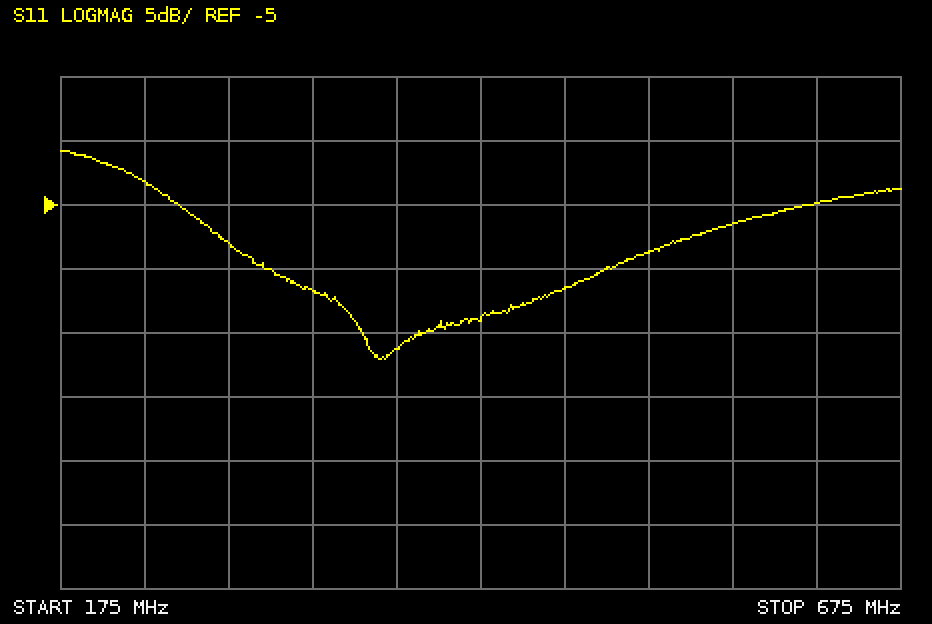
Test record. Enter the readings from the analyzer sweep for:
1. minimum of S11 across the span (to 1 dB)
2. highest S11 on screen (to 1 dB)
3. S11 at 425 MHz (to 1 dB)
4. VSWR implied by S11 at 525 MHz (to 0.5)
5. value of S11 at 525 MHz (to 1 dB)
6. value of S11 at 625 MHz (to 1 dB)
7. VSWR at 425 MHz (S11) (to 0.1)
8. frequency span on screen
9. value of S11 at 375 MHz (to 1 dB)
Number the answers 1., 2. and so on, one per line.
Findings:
1. -17 dB
2. -1 dB
3. -14 dB
4. 2.0
5. -9 dB
6. -5 dB
7. 1.5
8. 500 MHz
9. -16 dB
